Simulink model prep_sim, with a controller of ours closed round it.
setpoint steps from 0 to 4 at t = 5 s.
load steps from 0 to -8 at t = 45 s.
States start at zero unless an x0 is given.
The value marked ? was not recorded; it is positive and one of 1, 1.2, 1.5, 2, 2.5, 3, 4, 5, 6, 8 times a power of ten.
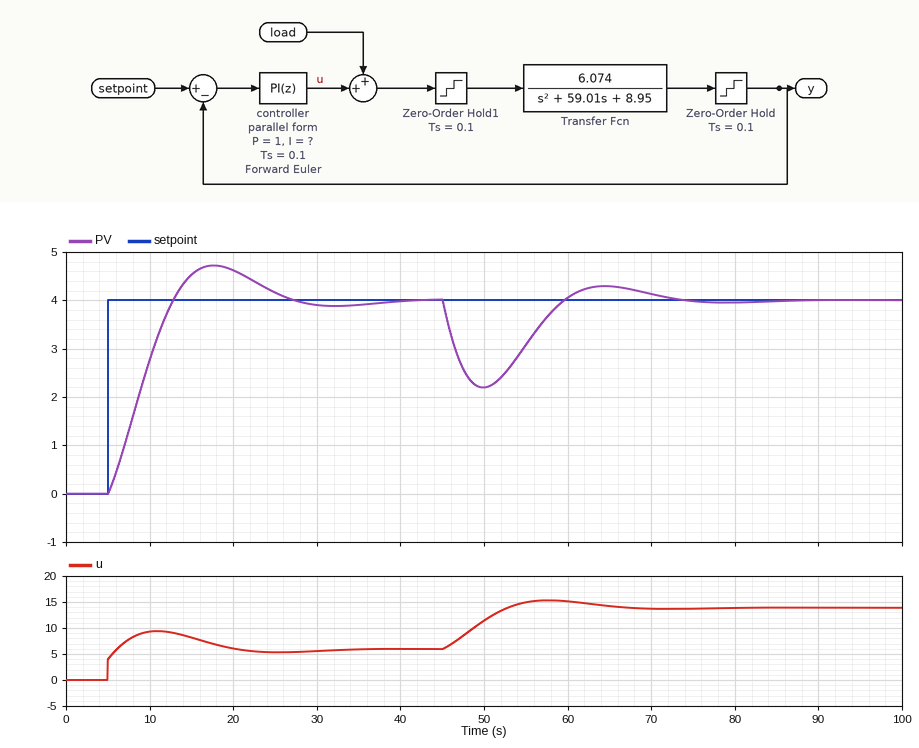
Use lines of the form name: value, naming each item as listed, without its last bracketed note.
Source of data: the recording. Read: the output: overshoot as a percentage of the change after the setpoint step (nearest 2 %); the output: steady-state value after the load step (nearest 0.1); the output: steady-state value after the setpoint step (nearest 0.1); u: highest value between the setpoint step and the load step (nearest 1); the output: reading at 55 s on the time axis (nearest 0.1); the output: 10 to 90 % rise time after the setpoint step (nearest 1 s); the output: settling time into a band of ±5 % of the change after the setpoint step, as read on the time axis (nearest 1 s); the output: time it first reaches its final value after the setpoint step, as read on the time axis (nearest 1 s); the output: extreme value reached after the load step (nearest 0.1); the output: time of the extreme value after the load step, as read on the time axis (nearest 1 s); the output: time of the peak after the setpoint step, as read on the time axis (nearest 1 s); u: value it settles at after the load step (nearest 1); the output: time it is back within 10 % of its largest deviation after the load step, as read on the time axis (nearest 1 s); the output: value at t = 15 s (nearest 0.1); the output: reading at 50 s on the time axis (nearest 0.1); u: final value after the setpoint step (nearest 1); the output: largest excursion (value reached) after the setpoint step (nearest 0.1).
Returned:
the output: overshoot as a percentage of the change after the setpoint step: 18 %
the output: steady-state value after the load step: 4.0
the output: steady-state value after the setpoint step: 4.0
u: highest value between the setpoint step and the load step: 9
the output: reading at 55 s on the time axis: 3.1
the output: 10 to 90 % rise time after the setpoint step: 6 s
the output: settling time into a band of ±5 % of the change after the setpoint step, as read on the time axis: 25 s
the output: time it first reaches its final value after the setpoint step, as read on the time axis: 13 s
the output: extreme value reached after the load step: 2.2
the output: time of the extreme value after the load step, as read on the time axis: 50 s
the output: time of the peak after the setpoint step, as read on the time axis: 18 s
u: value it settles at after the load step: 14
the output: time it is back within 10 % of its largest deviation after the load step, as read on the time axis: 69 s
the output: value at t = 15 s: 4.5
the output: reading at 50 s on the time axis: 2.2
u: final value after the setpoint step: 6
the output: largest excursion (value reached) after the setpoint step: 4.7
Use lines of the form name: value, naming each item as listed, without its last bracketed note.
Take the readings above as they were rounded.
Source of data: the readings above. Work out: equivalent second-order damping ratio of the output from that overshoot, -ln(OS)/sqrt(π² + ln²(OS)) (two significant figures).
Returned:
equivalent second-order damping ratio of the output from that overshoot, -ln(OS)/sqrt(π² + ln²(OS)): 0.48
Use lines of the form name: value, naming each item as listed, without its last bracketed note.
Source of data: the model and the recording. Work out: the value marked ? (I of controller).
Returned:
the value marked ?: 0.6
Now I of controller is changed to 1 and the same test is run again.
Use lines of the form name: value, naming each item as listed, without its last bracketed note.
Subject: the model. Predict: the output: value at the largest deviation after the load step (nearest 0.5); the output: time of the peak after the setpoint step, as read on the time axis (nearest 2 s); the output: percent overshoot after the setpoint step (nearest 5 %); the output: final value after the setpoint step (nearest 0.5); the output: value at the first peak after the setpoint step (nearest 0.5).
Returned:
the output: value at the largest deviation after the load step: 2.5
the output: time of the peak after the setpoint step, as read on the time axis: 14 s
the output: percent overshoot after the setpoint step: 30 %
the output: final value after the setpoint step: 4.0
the output: value at the first peak after the setpoint step: 5.0
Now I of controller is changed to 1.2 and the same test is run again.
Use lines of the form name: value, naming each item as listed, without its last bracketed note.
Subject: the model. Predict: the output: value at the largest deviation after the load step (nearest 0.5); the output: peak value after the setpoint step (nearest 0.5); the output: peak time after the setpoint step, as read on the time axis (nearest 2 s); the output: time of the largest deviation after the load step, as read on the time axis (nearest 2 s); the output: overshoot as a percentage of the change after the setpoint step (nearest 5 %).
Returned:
the output: value at the largest deviation after the load step: 2.5
the output: peak value after the setpoint step: 5.5
the output: peak time after the setpoint step, as read on the time axis: 14 s
the output: time of the largest deviation after the load step, as read on the time axis: 48 s
the output: overshoot as a percentage of the change after the setpoint step: 35 %
